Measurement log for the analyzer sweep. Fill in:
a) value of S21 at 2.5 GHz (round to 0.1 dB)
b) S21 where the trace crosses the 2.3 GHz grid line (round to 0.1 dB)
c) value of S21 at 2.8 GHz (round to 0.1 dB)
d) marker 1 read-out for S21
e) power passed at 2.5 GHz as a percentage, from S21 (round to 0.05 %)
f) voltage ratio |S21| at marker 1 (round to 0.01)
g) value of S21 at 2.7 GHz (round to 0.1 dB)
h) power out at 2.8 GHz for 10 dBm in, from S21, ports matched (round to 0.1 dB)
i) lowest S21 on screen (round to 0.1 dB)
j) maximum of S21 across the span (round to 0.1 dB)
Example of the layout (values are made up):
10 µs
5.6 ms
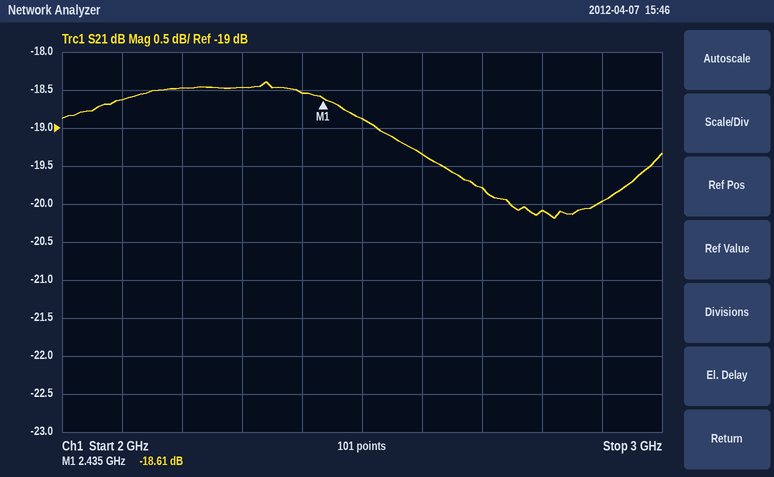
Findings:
-18.9 dB
-18.5 dB
-20.1 dB
-18.61 dB
1.30 %
0.12
-19.8 dB
-10.1 dBm
-20.2 dB
-18.4 dB
